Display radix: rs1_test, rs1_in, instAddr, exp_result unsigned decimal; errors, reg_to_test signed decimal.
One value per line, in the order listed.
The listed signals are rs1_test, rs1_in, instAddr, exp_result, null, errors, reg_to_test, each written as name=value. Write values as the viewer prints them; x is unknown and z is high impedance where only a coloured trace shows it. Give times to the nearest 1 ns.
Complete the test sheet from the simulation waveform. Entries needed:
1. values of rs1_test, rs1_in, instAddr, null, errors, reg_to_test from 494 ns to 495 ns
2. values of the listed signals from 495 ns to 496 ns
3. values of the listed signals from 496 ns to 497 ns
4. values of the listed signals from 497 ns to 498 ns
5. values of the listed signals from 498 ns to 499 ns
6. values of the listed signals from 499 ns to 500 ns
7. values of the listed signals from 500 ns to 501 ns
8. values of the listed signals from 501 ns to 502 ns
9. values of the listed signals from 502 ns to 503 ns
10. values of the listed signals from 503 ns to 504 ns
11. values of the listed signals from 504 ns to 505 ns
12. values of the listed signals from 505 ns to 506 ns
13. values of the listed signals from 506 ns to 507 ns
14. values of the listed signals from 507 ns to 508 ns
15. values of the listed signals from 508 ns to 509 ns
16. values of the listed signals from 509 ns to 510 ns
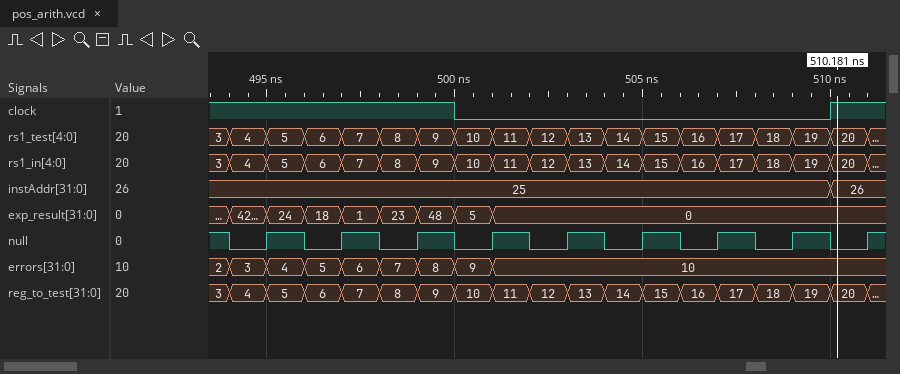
rs1_test=4, rs1_in=4, instAddr=25, null=0, errors=3, reg_to_test=4
rs1_test=5, rs1_in=5, instAddr=25, exp_result=24, null=1, errors=4, reg_to_test=5
rs1_test=6, rs1_in=6, instAddr=25, exp_result=18, null=0, errors=5, reg_to_test=6
rs1_test=7, rs1_in=7, instAddr=25, exp_result=1, null=1, errors=6, reg_to_test=7
rs1_test=8, rs1_in=8, instAddr=25, exp_result=23, null=0, errors=7, reg_to_test=8
rs1_test=9, rs1_in=9, instAddr=25, exp_result=48, null=1, errors=8, reg_to_test=9
rs1_test=10, rs1_in=10, instAddr=25, exp_result=5, null=0, errors=9, reg_to_test=10
rs1_test=11, rs1_in=11, instAddr=25, exp_result=0, null=1, errors=10, reg_to_test=11
rs1_test=12, rs1_in=12, instAddr=25, exp_result=0, null=0, errors=10, reg_to_test=12
rs1_test=13, rs1_in=13, instAddr=25, exp_result=0, null=1, errors=10, reg_to_test=13
rs1_test=14, rs1_in=14, instAddr=25, exp_result=0, null=0, errors=10, reg_to_test=14
rs1_test=15, rs1_in=15, instAddr=25, exp_result=0, null=1, errors=10, reg_to_test=15
rs1_test=16, rs1_in=16, instAddr=25, exp_result=0, null=0, errors=10, reg_to_test=16
rs1_test=17, rs1_in=17, instAddr=25, exp_result=0, null=1, errors=10, reg_to_test=17
rs1_test=18, rs1_in=18, instAddr=25, exp_result=0, null=0, errors=10, reg_to_test=18
rs1_test=19, rs1_in=19, instAddr=25, exp_result=0, null=1, errors=10, reg_to_test=19
